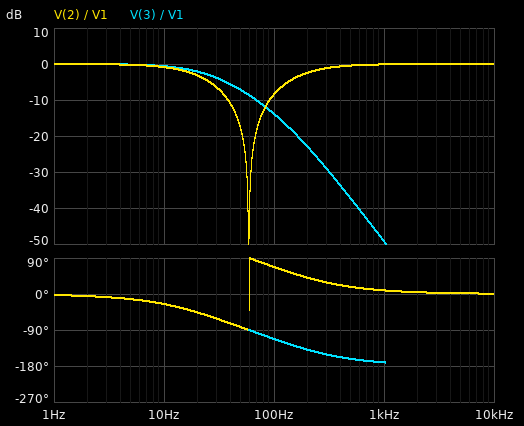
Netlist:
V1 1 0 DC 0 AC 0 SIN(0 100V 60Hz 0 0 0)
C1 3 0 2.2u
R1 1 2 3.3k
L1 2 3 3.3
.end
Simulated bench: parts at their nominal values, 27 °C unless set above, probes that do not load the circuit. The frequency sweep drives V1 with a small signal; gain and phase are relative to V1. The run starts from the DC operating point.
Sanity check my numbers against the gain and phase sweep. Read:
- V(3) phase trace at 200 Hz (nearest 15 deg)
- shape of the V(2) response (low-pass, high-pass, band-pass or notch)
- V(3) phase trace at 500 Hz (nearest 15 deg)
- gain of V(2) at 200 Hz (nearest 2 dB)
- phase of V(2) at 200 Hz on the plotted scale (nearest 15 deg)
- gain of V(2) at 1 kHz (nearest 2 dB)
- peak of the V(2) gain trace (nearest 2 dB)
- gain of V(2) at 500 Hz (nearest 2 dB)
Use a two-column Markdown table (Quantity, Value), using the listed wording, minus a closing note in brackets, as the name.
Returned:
| Quantity | Value |
|---|---|
| V(3) phase trace at 200 Hz | -135 deg |
| shape of the V(2) response | notch |
| V(3) phase trace at 500 Hz | -165 deg |
| gain of V(2) at 200 Hz | -2 dB |
| phase of V(2) at 200 Hz on the plotted scale | 45 deg |
| gain of V(2) at 1 kHz | 0 dB |
| peak of the V(2) gain trace | 0 dB |
| gain of V(2) at 500 Hz | 0 dB |
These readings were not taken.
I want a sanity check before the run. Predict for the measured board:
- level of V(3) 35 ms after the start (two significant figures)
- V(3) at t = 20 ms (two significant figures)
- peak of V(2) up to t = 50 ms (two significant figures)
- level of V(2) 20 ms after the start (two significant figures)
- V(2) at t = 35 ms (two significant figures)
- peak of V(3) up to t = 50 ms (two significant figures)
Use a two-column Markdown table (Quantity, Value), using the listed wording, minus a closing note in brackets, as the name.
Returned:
| Quantity | Value |
|---|---|
| level of V(3) 35 ms after the start | -30 V |
| V(3) at t = 20 ms | -10 V |
| peak of V(2) up to t = 50 ms | 30 V |
| level of V(2) 20 ms after the start | 2.4 V |
| V(2) at t = 35 ms | 1.1 V |
| peak of V(3) up to t = 50 ms | 48 V |
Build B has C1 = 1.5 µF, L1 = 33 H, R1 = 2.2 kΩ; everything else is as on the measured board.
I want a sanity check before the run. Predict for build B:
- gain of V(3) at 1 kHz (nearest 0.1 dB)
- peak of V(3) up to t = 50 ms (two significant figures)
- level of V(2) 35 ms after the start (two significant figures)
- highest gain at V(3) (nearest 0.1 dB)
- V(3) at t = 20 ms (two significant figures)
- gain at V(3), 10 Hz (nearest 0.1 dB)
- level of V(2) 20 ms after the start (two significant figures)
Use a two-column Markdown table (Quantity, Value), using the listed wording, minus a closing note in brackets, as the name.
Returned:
| Quantity | Value |
|---|---|
| gain of V(3) at 1 kHz | -65.8 dB |
| peak of V(3) up to t = 50 ms | 46 V |
| level of V(2) 35 ms after the start | 70 V |
| highest gain at V(3) | 6.8 dB |
| V(3) at t = 20 ms | -9.3 V |
| gain at V(3), 10 Hz | 1.6 dB |
| level of V(2) 20 ms after the start | 110 V |
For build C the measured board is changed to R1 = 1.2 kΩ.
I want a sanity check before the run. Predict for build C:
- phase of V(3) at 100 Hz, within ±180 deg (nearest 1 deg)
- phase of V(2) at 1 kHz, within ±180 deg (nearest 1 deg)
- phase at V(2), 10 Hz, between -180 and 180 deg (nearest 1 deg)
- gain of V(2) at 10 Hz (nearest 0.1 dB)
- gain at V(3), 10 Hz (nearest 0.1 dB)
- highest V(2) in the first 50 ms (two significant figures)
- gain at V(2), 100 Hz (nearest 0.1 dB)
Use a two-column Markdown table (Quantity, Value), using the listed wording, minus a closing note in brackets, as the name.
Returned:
| Quantity | Value |
|---|---|
| phase of V(3) at 100 Hz, within ±180 deg | -138 deg |
| phase of V(2) at 1 kHz, within ±180 deg | 3 deg |
| phase at V(2), 10 Hz, between -180 and 180 deg | -10 deg |
| gain of V(2) at 10 Hz | -0.1 dB |
| gain at V(3), 10 Hz | 0.1 dB |
| highest V(2) in the first 50 ms | 55 V |
| gain at V(2), 100 Hz | -2.5 dB |
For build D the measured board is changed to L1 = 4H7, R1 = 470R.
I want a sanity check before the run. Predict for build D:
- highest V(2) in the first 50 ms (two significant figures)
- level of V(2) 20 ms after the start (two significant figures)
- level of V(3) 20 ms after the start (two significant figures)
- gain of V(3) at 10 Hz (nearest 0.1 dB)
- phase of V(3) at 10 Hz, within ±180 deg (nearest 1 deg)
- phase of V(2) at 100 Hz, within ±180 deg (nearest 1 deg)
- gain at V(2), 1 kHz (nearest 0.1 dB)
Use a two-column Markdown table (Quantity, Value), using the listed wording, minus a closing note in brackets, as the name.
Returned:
| Quantity | Value |
|---|---|
| highest V(2) in the first 50 ms | 81 V |
| level of V(2) 20 ms after the start | 51 V |
| level of V(3) 20 ms after the start | -120 V |
| gain of V(3) at 10 Hz | 0.3 dB |
| phase of V(3) at 10 Hz, within ±180 deg | -4 deg |
| phase of V(2) at 100 Hz, within ±180 deg | 12 deg |
| gain at V(2), 1 kHz | 0 dB |
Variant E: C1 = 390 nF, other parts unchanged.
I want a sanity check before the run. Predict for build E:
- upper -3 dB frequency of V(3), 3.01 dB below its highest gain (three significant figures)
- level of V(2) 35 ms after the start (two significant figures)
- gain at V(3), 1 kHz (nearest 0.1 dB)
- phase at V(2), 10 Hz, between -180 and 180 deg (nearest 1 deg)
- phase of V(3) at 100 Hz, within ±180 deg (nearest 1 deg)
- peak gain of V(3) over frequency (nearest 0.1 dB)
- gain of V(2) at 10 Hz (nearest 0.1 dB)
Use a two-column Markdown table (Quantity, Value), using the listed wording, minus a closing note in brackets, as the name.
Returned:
| Quantity | Value |
|---|---|
| upper -3 dB frequency of V(3), 3.01 dB below its highest gain | 159 Hz |
| level of V(2) 35 ms after the start | 7.9 V |
| gain at V(3), 1 kHz | -34.1 dB |
| phase at V(2), 10 Hz, between -180 and 180 deg | -5 deg |
| phase of V(3) at 100 Hz, within ±180 deg | -59 deg |
| peak gain of V(3) over frequency | 0.6 dB |
| gain of V(2) at 10 Hz | 0 dB |
